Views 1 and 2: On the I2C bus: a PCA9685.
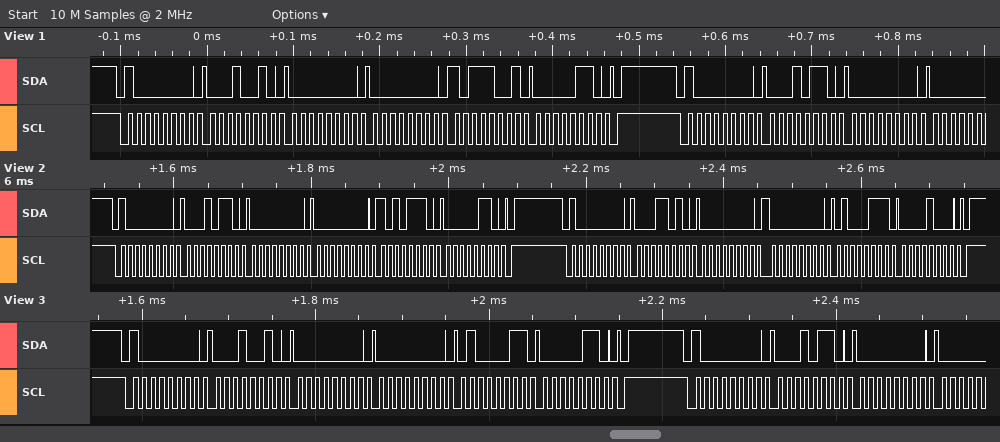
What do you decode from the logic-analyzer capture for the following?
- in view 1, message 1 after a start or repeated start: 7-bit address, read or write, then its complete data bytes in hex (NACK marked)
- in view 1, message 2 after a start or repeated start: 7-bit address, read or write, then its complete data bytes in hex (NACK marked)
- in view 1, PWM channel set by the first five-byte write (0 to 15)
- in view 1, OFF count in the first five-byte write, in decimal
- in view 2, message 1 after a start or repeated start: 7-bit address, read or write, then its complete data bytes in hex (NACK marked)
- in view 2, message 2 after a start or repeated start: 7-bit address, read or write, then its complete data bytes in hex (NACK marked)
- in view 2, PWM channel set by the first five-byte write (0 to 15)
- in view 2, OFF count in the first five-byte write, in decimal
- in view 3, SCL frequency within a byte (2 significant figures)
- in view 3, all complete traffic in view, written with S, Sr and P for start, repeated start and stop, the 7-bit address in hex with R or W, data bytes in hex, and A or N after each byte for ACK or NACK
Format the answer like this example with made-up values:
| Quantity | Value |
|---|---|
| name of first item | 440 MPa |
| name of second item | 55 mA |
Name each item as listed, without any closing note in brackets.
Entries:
| Quantity | Value |
|---|---|
| in view 1, message 1 after a start or repeated start: 7-bit address, read or write, then its complete data bytes in hex | 0x40 write: 12 00 00 B9 06 |
| in view 1, message 2 after a start or repeated start: 7-bit address, read or write, then its complete data bytes in hex | 0x40 write: 16 00 |
| in view 1, PWM channel set by the first five-byte write | 3 |
| in view 1, OFF count in the first five-byte write, in decimal | 1721 |
| in view 2, message 1 after a start or repeated start: 7-bit address, read or write, then its complete data bytes in hex | 0x40 write: 16 00 00 AE 06 |
| in view 2, message 2 after a start or repeated start: 7-bit address, read or write, then its complete data bytes in hex | 0x40 write: 1A 00 00 47 08 |
| in view 2, PWM channel set by the first five-byte write | 4 |
| in view 2, OFF count in the first five-byte write, in decimal | 1710 |
| in view 3, SCL frequency within a byte | 100 kHz |
| in view 3, all complete traffic in view, written with S, Sr and P for start, repeated start and stop, the 7-bit address in hex with R or W, data bytes in hex, and A or N after each byte for ACK or NACK | S 40W A 12 A 00 A 00 A 43 A 06 A P S 40W A 16 A 00 A |
